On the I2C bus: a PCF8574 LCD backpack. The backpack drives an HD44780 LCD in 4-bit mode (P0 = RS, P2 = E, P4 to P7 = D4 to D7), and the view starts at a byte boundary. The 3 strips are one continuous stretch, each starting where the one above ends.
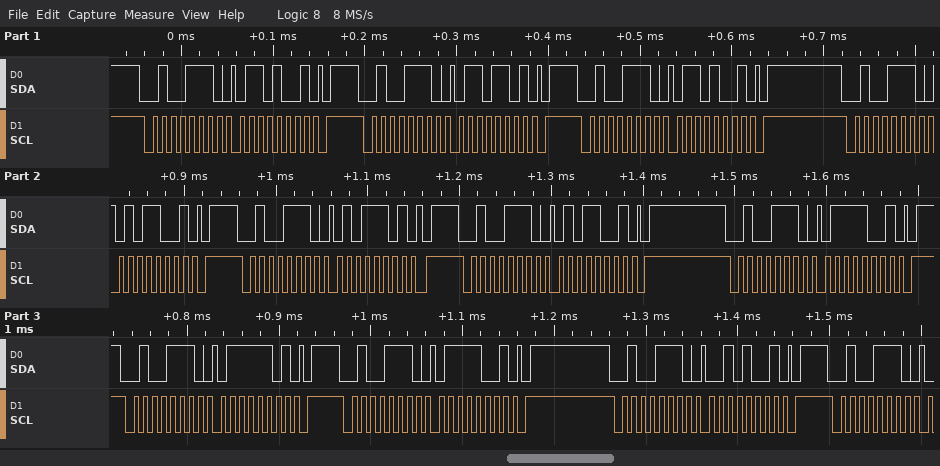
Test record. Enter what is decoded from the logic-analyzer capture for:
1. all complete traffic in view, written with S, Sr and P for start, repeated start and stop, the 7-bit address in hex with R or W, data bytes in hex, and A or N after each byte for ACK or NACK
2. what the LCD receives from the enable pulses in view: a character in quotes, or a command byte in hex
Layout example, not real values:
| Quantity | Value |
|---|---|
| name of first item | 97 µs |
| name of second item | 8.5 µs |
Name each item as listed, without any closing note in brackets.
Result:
| Quantity | Value |
|---|---|
| all complete traffic in view, written with S, Sr and P for start, repeated start and stop, the 7-bit address in hex with R or W, data bytes in hex, and A or N after each byte for ACK or NACK | S 27W A 69 A P S 27W A 6D A P S 27W A 69 A P S 27W A 59 A P S 27W A 5D A P S 27W A 59 A P S 27W A 79 A P S 27W A 7D A P S 27W A 79 A P S 27W A 29 A P S 27W A |
| what the LCD receives from the enable pulses in view: a character in quotes, or a command byte in hex | 'e' |
